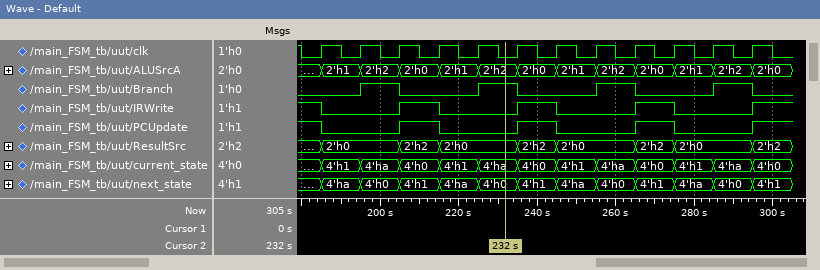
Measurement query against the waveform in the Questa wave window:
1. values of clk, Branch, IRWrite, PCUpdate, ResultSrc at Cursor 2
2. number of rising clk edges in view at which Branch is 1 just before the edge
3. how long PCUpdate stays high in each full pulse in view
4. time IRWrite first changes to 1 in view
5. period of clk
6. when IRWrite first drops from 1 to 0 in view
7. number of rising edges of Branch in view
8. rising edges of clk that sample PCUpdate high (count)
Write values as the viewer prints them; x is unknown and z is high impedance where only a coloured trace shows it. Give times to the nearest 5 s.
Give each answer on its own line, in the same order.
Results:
clk=0, Branch=1, IRWrite=0, PCUpdate=0, ResultSrc=2'h0
4
10 s, 10 s, 10 s
205 s
10 s
185 s
4
4
